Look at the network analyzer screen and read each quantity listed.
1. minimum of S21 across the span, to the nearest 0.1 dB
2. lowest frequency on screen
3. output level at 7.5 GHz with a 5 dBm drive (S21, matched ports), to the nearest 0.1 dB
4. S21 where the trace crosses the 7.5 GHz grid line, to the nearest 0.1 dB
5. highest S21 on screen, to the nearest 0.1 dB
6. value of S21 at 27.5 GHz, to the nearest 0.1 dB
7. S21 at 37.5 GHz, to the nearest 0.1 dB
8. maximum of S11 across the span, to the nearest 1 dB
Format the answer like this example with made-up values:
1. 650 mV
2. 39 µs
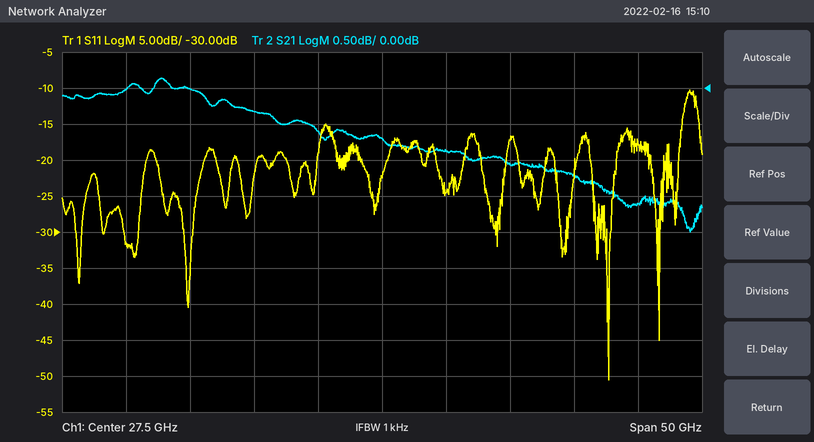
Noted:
1. -2.0 dB
2. 2.5 GHz
3. 5.0 dBm
4. 0.0 dB
5. 0.1 dB
6. -0.7 dB
7. -1.1 dB
8. -10 dB
